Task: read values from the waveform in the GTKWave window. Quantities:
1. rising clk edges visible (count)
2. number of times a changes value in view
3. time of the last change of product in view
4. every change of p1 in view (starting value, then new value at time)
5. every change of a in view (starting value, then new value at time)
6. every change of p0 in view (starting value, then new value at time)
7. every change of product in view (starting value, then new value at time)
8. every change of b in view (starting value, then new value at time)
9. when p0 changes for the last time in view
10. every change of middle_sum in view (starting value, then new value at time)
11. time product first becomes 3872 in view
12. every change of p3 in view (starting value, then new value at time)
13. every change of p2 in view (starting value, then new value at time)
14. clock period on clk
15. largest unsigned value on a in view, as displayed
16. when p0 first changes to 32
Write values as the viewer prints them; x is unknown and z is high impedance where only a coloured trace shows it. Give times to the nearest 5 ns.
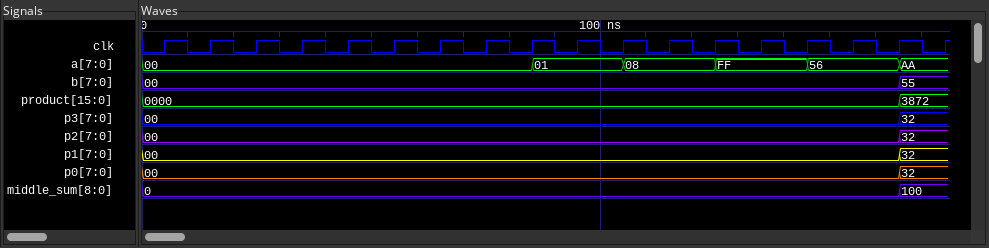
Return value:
18
5
165 ns
00, 32 at 165 ns
00, 01 at 85 ns, 08 at 105 ns, FF at 125 ns, 56 at 145 ns, AA at 165 ns
00, 32 at 165 ns
0000, 3872 at 165 ns
00, 55 at 165 ns
165 ns
0, 100 at 165 ns
165 ns
00, 32 at 165 ns
00, 32 at 165 ns
10 ns
FF
165 ns
